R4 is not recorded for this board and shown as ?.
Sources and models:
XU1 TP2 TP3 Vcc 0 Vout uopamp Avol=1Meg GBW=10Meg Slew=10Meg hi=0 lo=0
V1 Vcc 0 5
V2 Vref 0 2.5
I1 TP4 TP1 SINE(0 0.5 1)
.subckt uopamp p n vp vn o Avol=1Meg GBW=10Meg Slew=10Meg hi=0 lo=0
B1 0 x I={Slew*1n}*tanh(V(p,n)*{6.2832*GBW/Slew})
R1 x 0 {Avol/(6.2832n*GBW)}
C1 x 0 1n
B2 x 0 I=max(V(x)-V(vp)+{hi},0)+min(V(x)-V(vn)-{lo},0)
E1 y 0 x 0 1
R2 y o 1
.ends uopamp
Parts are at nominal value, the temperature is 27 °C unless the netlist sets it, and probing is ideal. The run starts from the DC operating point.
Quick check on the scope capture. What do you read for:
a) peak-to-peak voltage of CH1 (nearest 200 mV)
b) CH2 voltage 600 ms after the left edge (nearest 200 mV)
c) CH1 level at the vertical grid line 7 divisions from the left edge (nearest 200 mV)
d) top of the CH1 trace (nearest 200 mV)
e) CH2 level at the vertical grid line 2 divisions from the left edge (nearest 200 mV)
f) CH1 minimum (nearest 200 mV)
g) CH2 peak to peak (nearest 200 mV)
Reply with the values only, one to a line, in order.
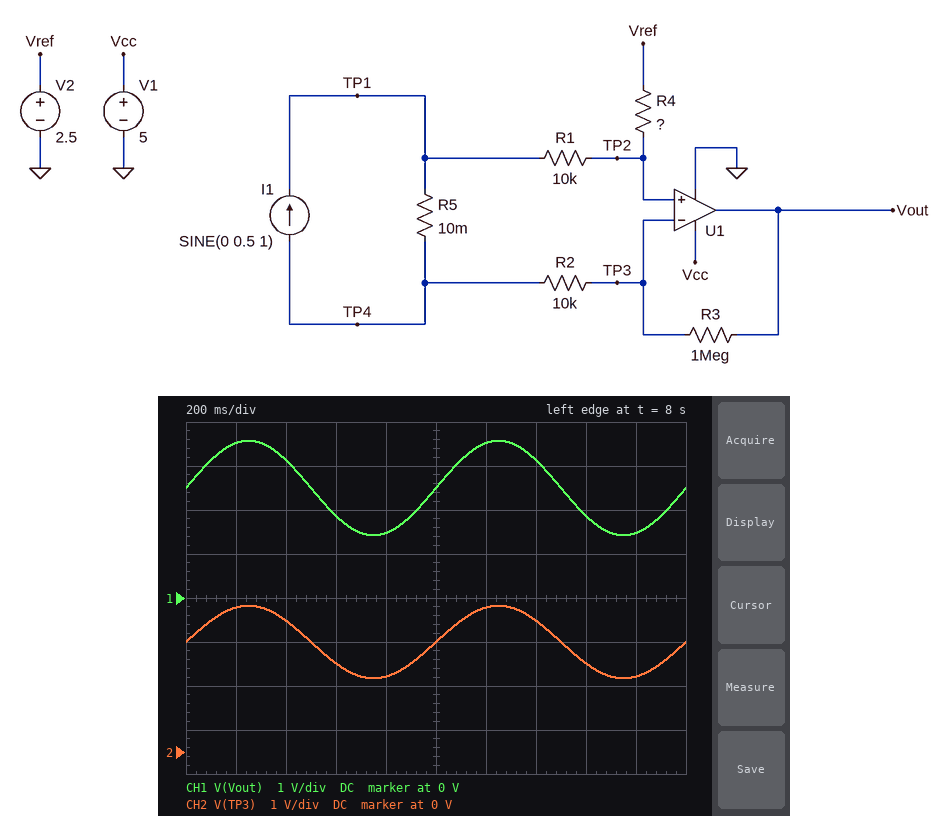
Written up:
2.2 V
2.0 V
3.2 V
3.6 V
3.0 V
1.4 V
1.6 V
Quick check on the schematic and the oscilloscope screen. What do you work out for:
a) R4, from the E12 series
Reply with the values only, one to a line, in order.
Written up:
3.3 MΩ
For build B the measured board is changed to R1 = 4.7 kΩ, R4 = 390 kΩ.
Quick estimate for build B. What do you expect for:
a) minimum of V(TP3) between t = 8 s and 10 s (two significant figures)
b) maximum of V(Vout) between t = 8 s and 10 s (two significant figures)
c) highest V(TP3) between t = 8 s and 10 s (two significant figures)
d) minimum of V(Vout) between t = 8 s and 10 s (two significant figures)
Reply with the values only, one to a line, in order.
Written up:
2.4 V
3.0 V
2.6 V
2.0 V
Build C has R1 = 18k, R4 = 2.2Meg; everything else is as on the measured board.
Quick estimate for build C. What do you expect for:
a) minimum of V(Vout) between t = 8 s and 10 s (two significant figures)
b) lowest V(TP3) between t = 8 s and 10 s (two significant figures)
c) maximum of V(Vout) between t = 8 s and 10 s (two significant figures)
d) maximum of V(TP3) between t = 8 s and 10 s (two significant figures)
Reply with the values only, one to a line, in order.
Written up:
1.9 V
2.1 V
3.1 V
2.9 V
